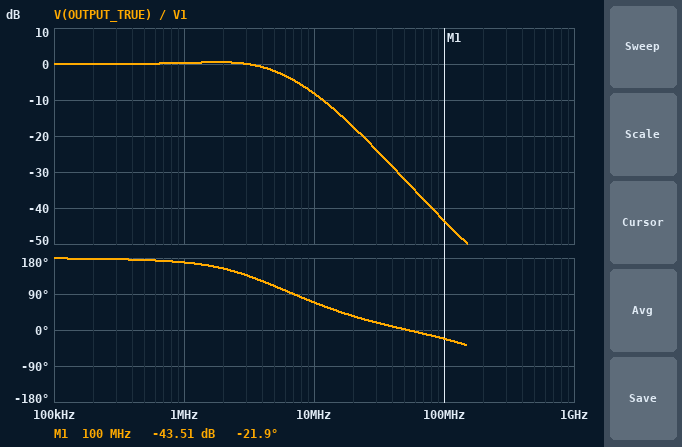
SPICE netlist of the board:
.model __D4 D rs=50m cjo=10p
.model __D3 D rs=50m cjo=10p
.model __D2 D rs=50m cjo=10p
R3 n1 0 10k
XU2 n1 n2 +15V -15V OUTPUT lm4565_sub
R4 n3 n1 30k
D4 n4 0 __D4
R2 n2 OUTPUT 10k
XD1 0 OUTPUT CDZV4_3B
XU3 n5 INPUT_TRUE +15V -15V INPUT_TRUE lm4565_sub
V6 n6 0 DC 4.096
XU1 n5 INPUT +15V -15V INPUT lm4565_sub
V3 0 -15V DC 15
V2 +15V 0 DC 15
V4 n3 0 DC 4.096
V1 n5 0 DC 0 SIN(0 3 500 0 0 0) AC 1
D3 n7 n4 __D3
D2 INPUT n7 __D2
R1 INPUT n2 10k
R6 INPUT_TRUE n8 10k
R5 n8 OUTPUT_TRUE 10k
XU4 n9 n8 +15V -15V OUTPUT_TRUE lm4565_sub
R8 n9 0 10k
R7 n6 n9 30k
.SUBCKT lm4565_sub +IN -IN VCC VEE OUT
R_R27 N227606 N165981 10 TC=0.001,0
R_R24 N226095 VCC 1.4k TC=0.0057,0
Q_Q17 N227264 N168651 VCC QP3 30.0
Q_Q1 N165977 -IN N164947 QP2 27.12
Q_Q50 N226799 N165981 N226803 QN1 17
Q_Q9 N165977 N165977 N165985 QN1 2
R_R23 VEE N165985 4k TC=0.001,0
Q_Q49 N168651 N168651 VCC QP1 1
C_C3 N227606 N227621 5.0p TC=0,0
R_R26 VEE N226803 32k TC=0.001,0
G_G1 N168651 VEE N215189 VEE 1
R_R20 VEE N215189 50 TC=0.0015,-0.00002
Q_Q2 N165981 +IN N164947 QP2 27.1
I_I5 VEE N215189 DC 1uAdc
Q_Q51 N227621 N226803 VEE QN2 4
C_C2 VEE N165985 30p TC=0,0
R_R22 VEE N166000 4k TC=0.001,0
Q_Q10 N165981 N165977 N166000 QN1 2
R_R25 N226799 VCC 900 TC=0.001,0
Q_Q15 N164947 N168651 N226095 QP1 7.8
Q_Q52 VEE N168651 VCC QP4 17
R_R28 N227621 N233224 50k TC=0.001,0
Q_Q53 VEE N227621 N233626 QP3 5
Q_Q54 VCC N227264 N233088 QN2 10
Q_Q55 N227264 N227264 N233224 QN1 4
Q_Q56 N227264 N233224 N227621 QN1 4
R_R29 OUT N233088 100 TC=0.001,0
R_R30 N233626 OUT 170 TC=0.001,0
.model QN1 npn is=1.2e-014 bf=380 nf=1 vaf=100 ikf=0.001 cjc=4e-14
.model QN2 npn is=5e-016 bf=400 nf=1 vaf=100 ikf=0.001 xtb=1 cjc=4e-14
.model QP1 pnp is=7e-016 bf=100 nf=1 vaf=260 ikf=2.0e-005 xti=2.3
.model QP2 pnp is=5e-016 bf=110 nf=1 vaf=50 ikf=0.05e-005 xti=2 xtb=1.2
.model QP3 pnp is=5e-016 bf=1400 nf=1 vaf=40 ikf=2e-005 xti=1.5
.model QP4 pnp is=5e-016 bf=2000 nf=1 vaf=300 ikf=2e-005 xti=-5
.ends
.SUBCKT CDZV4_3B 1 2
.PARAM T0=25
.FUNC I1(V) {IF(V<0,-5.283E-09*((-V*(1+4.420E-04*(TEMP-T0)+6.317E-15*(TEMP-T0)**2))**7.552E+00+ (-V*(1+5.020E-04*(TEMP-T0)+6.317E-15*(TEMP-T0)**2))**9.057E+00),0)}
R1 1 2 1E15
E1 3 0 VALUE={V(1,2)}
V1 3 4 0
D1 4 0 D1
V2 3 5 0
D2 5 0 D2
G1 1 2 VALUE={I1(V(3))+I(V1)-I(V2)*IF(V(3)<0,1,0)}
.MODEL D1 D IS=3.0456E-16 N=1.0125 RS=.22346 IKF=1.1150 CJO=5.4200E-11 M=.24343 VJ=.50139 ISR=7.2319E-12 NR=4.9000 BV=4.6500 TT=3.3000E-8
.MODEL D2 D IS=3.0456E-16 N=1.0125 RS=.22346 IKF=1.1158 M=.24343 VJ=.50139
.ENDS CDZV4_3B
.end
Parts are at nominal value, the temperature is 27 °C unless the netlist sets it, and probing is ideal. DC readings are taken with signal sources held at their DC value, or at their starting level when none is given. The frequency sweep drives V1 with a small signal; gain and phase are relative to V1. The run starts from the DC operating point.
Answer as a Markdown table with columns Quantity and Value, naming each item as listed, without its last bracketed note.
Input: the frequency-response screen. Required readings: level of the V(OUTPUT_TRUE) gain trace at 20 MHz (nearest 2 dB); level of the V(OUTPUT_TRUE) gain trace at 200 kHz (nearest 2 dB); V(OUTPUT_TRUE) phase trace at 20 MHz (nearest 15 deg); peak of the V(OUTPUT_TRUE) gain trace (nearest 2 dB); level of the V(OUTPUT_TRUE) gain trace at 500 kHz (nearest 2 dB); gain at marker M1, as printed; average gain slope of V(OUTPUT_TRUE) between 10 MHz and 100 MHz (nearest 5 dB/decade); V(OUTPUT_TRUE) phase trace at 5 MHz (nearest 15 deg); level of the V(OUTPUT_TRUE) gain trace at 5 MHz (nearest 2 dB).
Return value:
| Quantity | Value |
|---|---|
| level of the V(OUTPUT_TRUE) gain trace at 20 MHz | -18 dB |
| level of the V(OUTPUT_TRUE) gain trace at 200 kHz | 0 dB |
| V(OUTPUT_TRUE) phase trace at 20 MHz | 30 deg |
| peak of the V(OUTPUT_TRUE) gain trace | 0 dB |
| level of the V(OUTPUT_TRUE) gain trace at 500 kHz | 0 dB |
| gain at marker M1, as printed | -43.51 dB |
| average gain slope of V(OUTPUT_TRUE) between 10 MHz and 100 MHz | -35 dB/decade |
| V(OUTPUT_TRUE) phase trace at 5 MHz | 105 deg |
| level of the V(OUTPUT_TRUE) gain trace at 5 MHz | -2 dB |
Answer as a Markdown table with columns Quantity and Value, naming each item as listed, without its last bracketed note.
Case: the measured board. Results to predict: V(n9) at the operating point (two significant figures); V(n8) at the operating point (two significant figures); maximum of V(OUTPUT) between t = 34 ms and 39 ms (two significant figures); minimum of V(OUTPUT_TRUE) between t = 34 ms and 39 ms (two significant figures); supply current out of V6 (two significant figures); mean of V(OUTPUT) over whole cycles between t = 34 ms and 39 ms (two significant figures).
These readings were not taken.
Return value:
| Quantity | Value |
|---|---|
| V(n9) at the operating point | 1.0 V |
| V(n8) at the operating point | 1.0 V |
| maximum of V(OUTPUT) between t = 34 ms and 39 ms | 4.8 V |
| minimum of V(OUTPUT_TRUE) between t = 34 ms and 39 ms | -950 mV |
| supply current out of V6 | 100 µA |
| mean of V(OUTPUT) over whole cycles between t = 34 ms and 39 ms | 2.1 V |
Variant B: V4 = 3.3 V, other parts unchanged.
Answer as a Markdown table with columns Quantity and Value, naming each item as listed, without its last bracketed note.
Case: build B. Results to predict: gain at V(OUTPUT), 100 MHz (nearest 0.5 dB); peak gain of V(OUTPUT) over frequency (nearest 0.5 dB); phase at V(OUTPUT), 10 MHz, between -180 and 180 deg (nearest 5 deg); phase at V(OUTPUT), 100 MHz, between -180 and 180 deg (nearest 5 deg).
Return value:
| Quantity | Value |
|---|---|
| gain at V(OUTPUT), 100 MHz | -66.0 dB |
| peak gain of V(OUTPUT) over frequency | 1.5 dB |
| phase at V(OUTPUT), 10 MHz, between -180 and 180 deg | 15 deg |
| phase at V(OUTPUT), 100 MHz, between -180 and 180 deg | -165 deg |
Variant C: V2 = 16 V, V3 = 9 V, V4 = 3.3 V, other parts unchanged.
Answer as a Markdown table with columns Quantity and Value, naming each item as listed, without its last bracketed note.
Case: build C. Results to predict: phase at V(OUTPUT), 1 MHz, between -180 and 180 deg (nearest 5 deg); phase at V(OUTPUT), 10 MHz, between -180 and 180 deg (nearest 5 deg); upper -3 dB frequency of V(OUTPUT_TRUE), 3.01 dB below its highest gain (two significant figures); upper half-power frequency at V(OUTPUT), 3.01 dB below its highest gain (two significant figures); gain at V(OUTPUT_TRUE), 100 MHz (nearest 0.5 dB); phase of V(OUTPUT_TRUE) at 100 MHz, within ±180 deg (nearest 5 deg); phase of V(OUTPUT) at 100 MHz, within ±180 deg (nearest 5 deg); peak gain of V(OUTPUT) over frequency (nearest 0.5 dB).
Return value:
| Quantity | Value |
|---|---|
| phase at V(OUTPUT), 1 MHz, between -180 and 180 deg | 170 deg |
| phase at V(OUTPUT), 10 MHz, between -180 and 180 deg | 15 deg |
| upper -3 dB frequency of V(OUTPUT_TRUE), 3.01 dB below its highest gain | 5.3 MHz |
| upper half-power frequency at V(OUTPUT), 3.01 dB below its highest gain | 6.6 MHz |
| gain at V(OUTPUT_TRUE), 100 MHz | -44.0 dB |
| phase of V(OUTPUT_TRUE) at 100 MHz, within ±180 deg | -25 deg |
| phase of V(OUTPUT) at 100 MHz, within ±180 deg | -165 deg |
| peak gain of V(OUTPUT) over frequency | 1.5 dB |
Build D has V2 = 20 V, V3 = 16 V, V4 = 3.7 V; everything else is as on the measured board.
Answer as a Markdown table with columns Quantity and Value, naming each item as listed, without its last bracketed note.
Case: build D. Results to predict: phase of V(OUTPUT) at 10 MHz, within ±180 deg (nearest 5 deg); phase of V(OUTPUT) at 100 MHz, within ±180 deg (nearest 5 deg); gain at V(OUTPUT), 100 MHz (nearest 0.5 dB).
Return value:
| Quantity | Value |
|---|---|
| phase of V(OUTPUT) at 10 MHz, within ±180 deg | 20 deg |
| phase of V(OUTPUT) at 100 MHz, within ±180 deg | -160 deg |
| gain at V(OUTPUT), 100 MHz | -64.5 dB |
